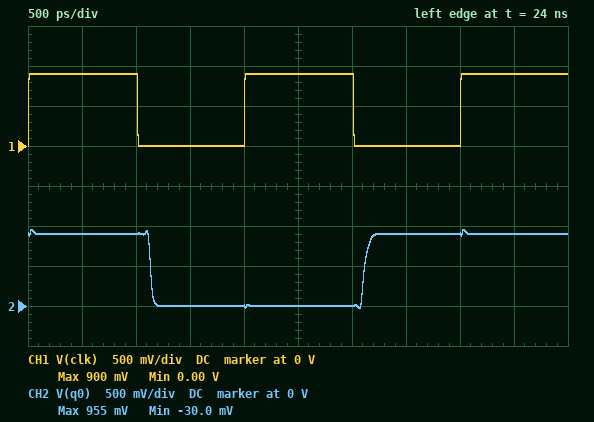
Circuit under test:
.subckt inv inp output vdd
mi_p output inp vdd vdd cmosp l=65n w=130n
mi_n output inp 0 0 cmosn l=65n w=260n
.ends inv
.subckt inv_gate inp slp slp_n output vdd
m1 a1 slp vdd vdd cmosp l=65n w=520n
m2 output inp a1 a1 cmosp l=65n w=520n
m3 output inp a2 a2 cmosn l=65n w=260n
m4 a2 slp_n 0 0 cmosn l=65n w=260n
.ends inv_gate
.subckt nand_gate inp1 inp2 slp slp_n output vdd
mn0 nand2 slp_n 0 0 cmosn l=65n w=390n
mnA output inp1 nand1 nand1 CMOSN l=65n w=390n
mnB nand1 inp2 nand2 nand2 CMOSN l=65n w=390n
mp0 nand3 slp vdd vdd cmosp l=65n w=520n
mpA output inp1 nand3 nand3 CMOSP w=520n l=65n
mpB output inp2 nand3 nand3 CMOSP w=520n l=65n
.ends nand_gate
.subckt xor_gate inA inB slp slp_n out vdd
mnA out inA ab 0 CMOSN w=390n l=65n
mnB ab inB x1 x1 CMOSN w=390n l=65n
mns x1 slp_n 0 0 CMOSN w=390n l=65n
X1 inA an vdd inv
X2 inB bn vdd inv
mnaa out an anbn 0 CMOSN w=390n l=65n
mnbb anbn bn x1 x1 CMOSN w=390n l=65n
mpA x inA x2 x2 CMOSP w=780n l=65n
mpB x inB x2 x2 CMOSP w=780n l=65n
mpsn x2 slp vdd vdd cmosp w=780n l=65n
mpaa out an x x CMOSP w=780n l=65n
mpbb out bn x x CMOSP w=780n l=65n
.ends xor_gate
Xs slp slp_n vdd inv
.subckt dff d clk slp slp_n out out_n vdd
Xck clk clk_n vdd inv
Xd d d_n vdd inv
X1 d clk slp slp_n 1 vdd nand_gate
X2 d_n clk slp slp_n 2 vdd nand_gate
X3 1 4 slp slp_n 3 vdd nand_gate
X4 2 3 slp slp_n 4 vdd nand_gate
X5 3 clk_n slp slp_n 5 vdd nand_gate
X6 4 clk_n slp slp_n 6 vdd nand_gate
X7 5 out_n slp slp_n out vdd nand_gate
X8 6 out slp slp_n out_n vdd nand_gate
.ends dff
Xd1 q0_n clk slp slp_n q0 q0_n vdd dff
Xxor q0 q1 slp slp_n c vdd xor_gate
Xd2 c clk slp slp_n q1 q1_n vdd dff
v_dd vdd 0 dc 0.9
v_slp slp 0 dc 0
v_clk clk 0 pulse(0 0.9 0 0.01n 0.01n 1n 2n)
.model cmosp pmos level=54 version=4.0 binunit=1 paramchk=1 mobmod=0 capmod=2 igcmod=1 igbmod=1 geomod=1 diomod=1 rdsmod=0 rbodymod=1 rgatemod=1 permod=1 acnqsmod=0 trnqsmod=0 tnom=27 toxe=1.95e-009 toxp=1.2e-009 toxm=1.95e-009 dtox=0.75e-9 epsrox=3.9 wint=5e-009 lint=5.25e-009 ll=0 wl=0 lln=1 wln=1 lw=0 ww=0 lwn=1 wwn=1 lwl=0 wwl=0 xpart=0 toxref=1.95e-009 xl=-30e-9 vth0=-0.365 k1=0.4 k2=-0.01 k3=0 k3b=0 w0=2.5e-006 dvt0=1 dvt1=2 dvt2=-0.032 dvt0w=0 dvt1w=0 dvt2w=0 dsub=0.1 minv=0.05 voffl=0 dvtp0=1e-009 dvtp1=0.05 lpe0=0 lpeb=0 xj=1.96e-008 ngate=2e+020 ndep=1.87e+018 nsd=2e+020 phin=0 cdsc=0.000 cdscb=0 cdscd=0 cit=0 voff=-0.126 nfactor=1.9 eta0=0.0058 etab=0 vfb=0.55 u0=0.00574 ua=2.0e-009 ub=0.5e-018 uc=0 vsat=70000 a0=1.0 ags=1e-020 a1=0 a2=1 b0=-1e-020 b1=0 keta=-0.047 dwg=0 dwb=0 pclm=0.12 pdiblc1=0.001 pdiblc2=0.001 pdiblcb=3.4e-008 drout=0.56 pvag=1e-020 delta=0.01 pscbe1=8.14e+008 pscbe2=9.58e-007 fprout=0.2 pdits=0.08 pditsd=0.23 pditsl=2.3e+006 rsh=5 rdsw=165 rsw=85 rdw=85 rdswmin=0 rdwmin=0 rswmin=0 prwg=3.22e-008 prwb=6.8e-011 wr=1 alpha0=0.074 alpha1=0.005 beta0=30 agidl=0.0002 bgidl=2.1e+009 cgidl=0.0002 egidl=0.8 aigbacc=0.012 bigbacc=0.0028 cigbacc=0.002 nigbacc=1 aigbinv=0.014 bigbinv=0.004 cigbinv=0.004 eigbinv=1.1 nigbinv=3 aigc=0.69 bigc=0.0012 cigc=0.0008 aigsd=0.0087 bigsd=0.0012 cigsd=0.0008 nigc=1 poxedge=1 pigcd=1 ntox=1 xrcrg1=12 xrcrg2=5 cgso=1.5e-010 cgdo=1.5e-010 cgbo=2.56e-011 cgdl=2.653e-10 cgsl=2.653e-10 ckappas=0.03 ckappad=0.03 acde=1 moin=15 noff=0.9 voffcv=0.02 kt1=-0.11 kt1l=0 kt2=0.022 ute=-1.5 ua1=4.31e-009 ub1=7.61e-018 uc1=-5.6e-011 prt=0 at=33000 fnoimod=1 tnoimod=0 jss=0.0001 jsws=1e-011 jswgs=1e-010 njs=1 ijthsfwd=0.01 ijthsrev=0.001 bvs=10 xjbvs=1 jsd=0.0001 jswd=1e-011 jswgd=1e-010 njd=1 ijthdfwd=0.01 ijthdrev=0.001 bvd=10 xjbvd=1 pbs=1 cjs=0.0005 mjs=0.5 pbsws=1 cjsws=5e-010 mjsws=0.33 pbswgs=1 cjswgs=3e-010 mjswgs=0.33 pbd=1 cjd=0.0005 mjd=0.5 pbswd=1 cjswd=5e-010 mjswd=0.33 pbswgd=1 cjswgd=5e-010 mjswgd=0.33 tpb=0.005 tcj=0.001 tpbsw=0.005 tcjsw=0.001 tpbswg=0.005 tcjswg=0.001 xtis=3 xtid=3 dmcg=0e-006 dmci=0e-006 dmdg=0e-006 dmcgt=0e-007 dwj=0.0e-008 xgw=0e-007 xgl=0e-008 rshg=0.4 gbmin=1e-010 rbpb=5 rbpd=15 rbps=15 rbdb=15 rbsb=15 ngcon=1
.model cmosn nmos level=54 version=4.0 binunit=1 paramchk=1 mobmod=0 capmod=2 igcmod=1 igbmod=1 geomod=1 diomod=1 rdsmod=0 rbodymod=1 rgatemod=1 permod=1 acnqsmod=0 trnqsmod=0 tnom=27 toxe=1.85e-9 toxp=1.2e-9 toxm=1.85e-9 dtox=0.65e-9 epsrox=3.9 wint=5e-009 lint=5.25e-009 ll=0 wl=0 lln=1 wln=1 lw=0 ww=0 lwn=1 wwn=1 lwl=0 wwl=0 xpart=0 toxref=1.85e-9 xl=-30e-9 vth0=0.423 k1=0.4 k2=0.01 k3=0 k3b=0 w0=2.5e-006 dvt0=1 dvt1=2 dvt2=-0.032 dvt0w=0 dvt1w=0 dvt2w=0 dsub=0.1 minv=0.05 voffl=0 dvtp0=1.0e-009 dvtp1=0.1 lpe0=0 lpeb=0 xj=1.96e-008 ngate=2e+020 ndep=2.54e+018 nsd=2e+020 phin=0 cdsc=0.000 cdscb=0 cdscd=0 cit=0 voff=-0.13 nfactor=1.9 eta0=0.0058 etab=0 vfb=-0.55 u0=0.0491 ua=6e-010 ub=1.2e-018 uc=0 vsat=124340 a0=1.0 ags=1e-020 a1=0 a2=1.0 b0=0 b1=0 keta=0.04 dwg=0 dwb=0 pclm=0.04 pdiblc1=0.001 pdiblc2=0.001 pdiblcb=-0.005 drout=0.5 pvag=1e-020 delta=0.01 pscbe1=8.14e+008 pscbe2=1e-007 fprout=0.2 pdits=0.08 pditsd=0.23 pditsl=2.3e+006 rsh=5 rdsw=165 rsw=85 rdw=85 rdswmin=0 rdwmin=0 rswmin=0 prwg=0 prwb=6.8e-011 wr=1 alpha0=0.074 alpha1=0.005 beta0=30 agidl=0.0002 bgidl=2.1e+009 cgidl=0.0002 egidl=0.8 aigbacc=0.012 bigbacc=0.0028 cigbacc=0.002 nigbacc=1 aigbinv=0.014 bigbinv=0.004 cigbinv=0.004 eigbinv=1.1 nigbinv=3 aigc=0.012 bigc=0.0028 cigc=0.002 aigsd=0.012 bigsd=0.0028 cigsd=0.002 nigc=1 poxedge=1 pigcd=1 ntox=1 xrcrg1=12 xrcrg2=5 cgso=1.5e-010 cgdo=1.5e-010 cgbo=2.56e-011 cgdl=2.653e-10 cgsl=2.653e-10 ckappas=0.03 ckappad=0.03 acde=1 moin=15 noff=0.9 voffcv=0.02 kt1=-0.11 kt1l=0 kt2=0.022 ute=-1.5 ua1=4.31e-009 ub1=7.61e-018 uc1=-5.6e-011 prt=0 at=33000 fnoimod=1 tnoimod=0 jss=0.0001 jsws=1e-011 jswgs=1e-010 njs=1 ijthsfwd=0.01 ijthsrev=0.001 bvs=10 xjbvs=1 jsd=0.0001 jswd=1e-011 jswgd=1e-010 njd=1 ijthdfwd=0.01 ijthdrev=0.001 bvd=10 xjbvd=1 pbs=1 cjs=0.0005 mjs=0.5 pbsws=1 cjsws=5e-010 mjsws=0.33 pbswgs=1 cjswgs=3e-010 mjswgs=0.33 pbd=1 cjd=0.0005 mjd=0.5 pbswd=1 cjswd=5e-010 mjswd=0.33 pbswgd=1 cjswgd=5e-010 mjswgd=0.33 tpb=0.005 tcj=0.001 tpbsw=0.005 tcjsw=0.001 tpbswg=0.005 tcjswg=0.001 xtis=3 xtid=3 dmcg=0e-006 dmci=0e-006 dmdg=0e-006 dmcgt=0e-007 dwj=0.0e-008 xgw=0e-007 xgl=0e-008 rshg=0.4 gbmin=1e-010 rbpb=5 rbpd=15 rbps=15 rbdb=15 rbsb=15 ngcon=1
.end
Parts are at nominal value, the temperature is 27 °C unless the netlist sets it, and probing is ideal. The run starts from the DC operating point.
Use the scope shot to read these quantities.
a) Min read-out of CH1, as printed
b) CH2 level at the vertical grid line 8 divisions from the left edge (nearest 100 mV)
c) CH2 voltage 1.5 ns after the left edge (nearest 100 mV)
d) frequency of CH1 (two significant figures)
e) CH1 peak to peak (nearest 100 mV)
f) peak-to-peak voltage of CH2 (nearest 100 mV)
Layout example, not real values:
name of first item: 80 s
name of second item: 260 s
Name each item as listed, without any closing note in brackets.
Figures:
Min read-out of CH1, as printed: 0.00 V
CH2 level at the vertical grid line 8 divisions from the left edge: 900 mV
CH2 voltage 1.5 ns after the left edge: 0 V
frequency of CH1: 500 MHz
CH1 peak to peak: 900 mV
peak-to-peak voltage of CH2: 1.0 V
